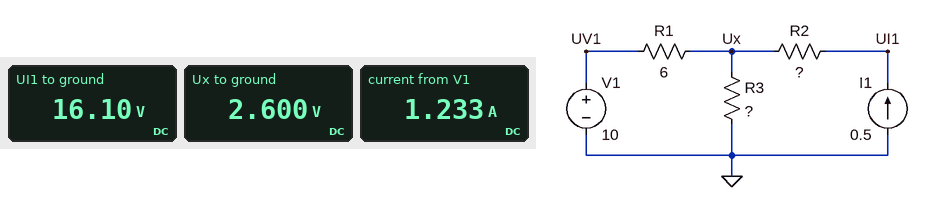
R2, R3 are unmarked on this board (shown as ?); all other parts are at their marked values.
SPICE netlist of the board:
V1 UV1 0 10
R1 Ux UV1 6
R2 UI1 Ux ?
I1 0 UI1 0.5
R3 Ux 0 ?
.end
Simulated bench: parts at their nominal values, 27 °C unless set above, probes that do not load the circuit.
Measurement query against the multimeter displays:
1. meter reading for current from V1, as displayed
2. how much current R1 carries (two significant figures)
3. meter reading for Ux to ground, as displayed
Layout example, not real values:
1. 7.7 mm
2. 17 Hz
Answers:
1. 1.233 A
2. 1.2 A
3. 2.600 V
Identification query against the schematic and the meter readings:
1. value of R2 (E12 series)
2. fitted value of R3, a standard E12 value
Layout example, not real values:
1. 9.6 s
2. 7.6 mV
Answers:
1. 27 Ω
2. 1.5 Ω
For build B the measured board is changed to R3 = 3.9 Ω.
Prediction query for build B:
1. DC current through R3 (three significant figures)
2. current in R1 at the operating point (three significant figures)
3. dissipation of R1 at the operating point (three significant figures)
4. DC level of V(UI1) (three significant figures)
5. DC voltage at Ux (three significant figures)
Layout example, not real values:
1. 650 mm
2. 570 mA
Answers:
1. 1.31 A
2. 813 mA
3. 3.97 W
4. 18.6 V
5. 5.12 V
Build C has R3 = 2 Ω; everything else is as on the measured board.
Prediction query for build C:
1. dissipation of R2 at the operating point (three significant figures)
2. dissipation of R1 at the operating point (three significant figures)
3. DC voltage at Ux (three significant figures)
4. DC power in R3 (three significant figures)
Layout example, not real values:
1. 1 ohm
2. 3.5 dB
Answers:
1. 6.75 W
2. 7.59 W
3. 3.25 V
4. 5.28 W
